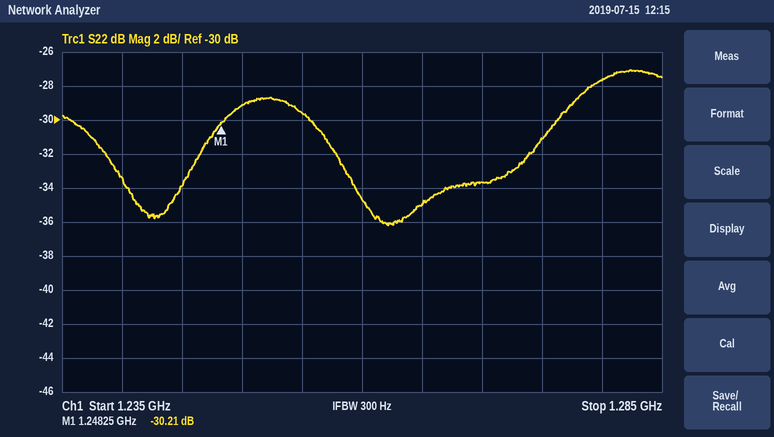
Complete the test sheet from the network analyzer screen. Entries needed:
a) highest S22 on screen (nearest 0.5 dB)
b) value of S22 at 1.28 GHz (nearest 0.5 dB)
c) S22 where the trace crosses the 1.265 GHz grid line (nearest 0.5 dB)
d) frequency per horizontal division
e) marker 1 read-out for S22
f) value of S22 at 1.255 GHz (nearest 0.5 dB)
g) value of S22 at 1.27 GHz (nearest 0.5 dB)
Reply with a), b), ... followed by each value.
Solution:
a) -27.0 dB
b) -27.5 dB
c) -35.0 dB
d) 5 MHz
e) -30.21 dB
f) -29.5 dB
g) -33.5 dB
